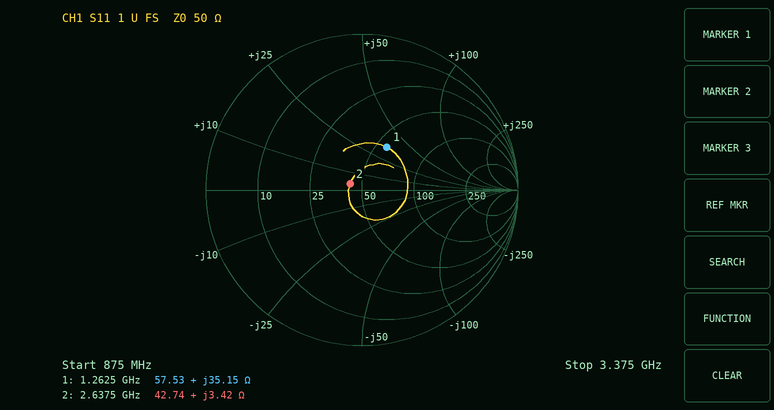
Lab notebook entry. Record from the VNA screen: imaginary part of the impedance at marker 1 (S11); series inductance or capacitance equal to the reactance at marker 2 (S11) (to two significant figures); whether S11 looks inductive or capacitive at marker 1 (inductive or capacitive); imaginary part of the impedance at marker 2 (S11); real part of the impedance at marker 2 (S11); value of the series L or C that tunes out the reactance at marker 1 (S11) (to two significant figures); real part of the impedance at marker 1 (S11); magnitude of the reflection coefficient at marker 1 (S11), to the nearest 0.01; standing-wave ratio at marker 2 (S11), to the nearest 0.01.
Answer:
+35.15 Ω
210 pH
inductive
+3.42 Ω
42.74 Ω
3.6 pF
57.53 Ω
0.32
1.19
